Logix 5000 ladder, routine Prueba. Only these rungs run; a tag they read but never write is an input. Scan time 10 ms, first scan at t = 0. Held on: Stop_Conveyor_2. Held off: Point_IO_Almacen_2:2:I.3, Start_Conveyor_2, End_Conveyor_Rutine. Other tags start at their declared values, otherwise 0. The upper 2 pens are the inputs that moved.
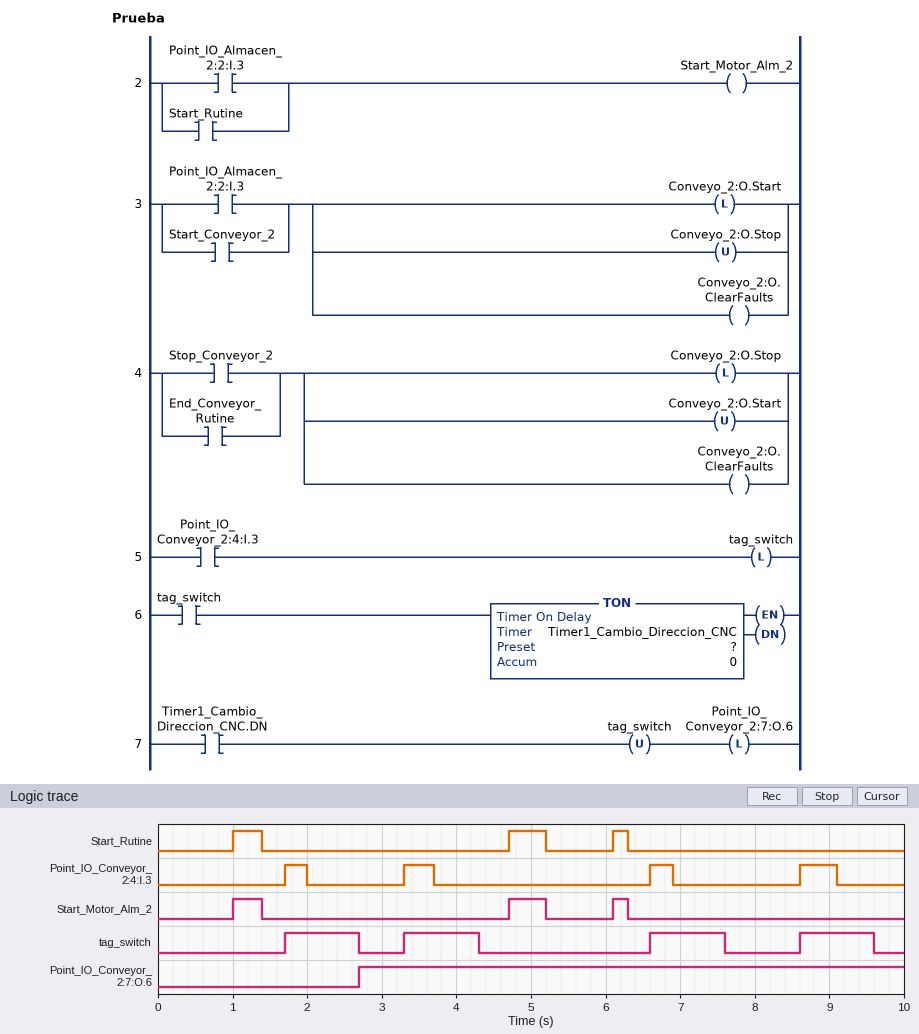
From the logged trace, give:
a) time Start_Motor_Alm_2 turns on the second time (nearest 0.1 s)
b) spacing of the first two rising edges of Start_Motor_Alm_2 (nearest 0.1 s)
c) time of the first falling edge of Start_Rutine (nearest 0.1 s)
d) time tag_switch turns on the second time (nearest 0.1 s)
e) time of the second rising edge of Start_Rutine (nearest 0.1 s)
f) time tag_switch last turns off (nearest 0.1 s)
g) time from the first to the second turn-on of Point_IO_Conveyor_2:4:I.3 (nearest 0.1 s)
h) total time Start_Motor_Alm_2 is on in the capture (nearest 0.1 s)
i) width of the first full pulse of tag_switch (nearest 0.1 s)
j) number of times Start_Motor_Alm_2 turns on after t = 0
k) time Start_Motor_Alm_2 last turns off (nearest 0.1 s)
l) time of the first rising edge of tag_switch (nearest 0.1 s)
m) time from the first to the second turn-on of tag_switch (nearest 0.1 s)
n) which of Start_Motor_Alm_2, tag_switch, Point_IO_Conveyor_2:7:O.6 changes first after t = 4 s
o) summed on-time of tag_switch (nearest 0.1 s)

4.7 s
3.7 s
1.4 s
3.3 s
4.7 s
9.6 s
1.6 s
1.1 s
1.0 s
3
6.3 s
1.7 s
1.6 s
tag_switch
4.0 s
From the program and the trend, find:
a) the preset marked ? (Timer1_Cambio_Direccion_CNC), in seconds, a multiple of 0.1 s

1.0 s
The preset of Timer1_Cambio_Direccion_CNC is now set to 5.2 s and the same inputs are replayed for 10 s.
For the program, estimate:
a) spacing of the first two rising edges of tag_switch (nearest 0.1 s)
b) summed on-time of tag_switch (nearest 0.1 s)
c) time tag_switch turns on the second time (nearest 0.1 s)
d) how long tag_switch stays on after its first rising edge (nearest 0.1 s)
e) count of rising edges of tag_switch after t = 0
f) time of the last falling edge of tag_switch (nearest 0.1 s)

6.9 s
6.6 s
8.6 s
5.2 s
2
6.9 s
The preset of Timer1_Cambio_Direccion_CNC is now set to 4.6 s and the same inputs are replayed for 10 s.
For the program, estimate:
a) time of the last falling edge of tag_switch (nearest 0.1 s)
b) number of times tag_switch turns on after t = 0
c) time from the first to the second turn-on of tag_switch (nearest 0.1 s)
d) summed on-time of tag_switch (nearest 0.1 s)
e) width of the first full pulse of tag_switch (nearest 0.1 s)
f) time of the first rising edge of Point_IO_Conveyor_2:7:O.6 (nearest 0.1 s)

6.3 s
2
4.9 s
8.0 s
4.6 s
6.3 s
